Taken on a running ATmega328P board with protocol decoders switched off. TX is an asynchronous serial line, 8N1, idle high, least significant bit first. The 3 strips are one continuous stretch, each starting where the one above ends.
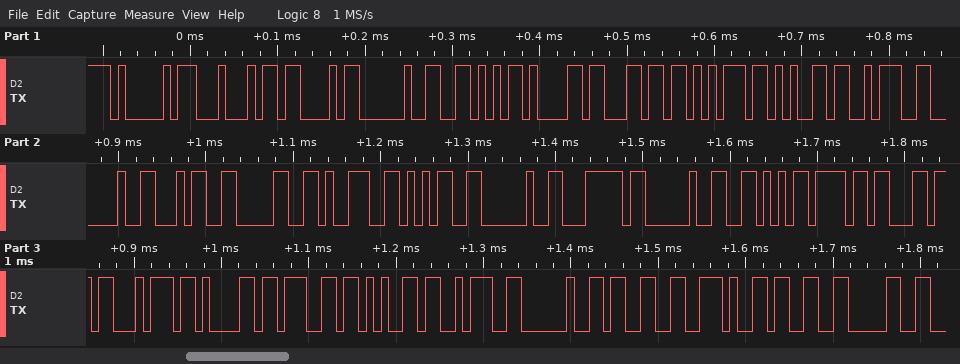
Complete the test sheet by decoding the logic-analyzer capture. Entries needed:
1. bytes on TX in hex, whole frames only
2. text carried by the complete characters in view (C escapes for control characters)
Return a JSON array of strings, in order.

["41 44 43 20 56 61 6C 75 65 3A 20 34 30 39 35 20 7C 20 56 6F 6C 74 61 67 65 3A 20 33 2E 33 30", "\"ADC Value: 4095 | Voltage: 3.30\""]
